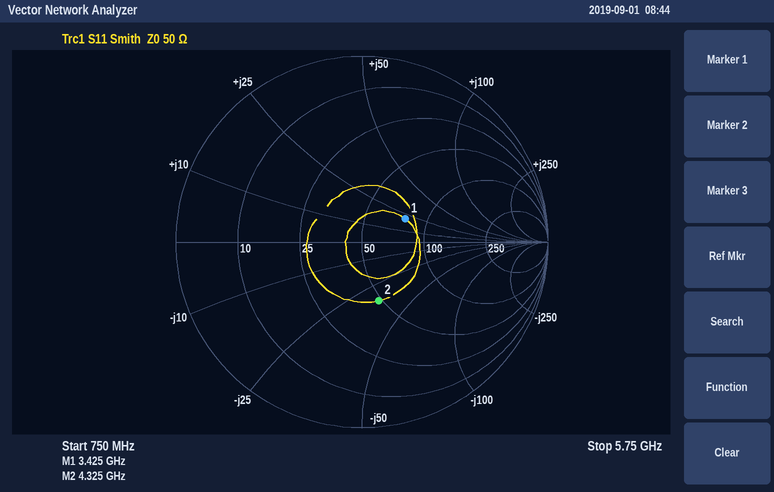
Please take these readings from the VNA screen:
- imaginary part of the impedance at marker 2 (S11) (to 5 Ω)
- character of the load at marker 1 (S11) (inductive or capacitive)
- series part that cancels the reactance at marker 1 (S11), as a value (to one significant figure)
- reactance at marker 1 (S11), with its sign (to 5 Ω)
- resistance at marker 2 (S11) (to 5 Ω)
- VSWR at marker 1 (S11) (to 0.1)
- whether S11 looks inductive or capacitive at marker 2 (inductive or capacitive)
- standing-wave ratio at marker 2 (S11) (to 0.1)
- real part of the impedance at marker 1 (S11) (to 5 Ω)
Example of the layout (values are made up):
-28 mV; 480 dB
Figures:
-35 Ω; inductive; 2 pF; +20 Ω; 50 Ω; 1.7; capacitive; 2.0; 75 Ω
